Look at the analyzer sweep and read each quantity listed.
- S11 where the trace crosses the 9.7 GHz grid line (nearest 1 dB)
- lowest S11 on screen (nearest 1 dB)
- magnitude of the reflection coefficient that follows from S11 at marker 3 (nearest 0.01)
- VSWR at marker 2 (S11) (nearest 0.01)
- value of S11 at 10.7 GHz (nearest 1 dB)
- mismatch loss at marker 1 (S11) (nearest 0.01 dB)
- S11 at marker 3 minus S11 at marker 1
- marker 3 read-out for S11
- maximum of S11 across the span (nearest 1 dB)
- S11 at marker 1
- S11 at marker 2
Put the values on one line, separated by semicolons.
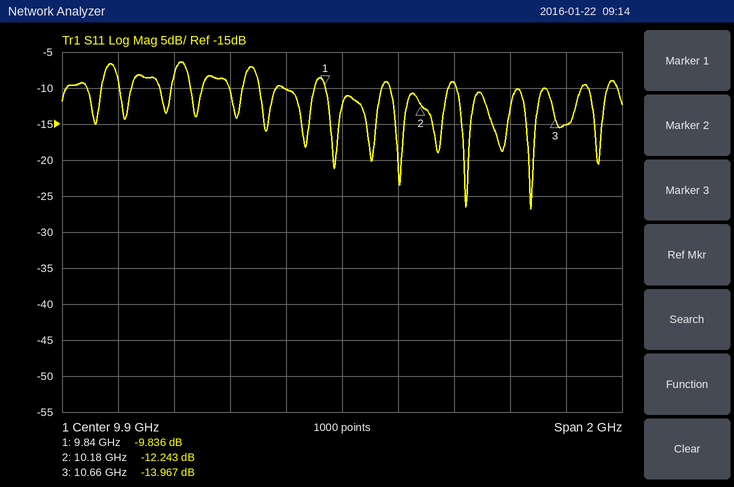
-10 dB; -27 dB; 0.20; 1.65; -15 dB; 0.48 dB; -4.131 dB; -13.967 dB; -6 dB; -9.836 dB; -12.243 dB
